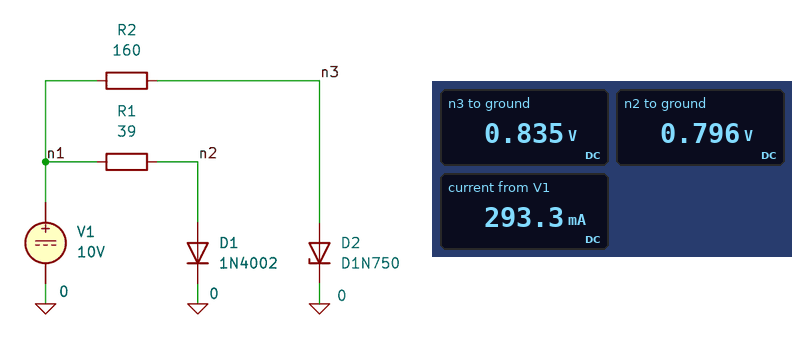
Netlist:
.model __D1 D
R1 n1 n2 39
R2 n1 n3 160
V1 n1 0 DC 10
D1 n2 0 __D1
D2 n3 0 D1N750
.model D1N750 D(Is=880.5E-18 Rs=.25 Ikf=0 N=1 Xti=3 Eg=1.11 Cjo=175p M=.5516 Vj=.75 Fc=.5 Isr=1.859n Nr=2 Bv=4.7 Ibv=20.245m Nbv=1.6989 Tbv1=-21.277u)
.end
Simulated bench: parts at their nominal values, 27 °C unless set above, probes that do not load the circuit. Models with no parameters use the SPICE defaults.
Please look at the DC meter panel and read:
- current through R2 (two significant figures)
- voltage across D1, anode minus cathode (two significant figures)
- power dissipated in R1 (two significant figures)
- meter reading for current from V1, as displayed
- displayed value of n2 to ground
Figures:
57 mA
800 mV
2.2 W
293.3 mA
0.796 V
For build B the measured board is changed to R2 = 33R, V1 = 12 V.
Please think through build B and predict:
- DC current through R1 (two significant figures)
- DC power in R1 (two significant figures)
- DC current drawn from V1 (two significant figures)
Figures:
290 mA
3.2 W
620 mA
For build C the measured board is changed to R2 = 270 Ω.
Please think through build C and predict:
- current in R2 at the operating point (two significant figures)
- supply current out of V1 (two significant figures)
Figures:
34 mA
270 mA
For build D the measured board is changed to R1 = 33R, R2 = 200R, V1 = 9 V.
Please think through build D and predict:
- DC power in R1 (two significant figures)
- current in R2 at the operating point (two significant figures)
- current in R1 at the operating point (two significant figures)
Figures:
2.0 W
41 mA
250 mA
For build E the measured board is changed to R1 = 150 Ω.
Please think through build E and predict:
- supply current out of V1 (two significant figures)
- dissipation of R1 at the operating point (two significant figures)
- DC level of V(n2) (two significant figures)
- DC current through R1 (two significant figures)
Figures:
120 mA
570 mW
760 mV
62 mA
